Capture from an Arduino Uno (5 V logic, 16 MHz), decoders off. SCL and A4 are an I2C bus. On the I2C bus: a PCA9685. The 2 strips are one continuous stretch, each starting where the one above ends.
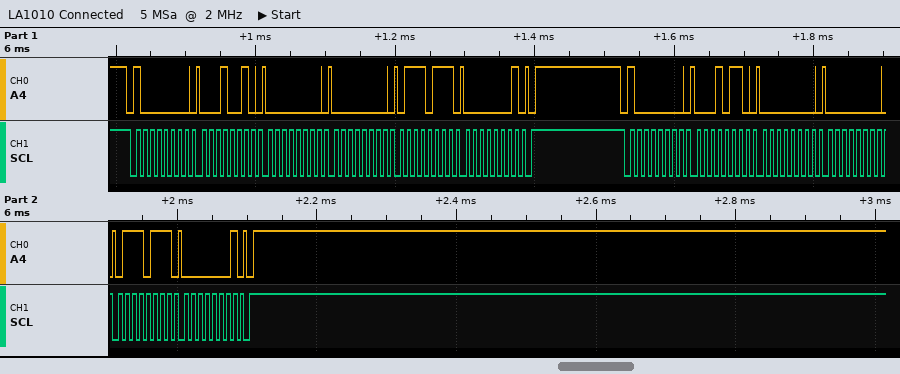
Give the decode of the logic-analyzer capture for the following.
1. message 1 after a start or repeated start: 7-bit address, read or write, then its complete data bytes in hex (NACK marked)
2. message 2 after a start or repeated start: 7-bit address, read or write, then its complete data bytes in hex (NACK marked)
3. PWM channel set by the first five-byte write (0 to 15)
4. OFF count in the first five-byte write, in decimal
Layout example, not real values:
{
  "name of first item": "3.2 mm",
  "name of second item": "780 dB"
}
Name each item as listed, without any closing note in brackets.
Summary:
{
  "message 1 after a start or repeated start: 7-bit address, read or write, then its complete data bytes in hex": "0x40 write: 12 00 00 77 01",
  "message 2 after a start or repeated start: 7-bit address, read or write, then its complete data bytes in hex": "0x40 write: 16 00 00 77 01",
  "PWM channel set by the first five-byte write": "3",
  "OFF count in the first five-byte write, in decimal": "375"
}
